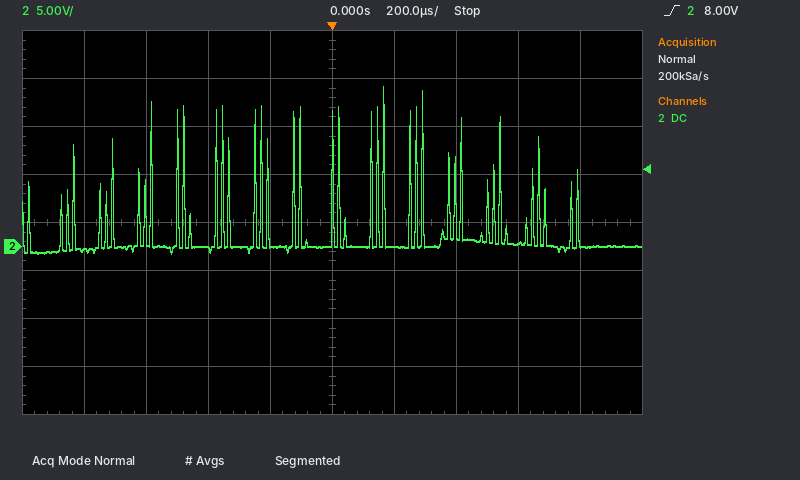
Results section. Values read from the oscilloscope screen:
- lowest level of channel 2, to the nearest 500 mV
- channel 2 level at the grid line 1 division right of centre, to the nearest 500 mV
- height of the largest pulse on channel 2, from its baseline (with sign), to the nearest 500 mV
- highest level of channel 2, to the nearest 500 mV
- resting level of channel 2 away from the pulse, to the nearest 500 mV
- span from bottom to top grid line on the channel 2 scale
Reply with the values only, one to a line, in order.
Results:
-500 mV
0.0 V
+16.5 V
16.5 V
0.0 V
40 V
